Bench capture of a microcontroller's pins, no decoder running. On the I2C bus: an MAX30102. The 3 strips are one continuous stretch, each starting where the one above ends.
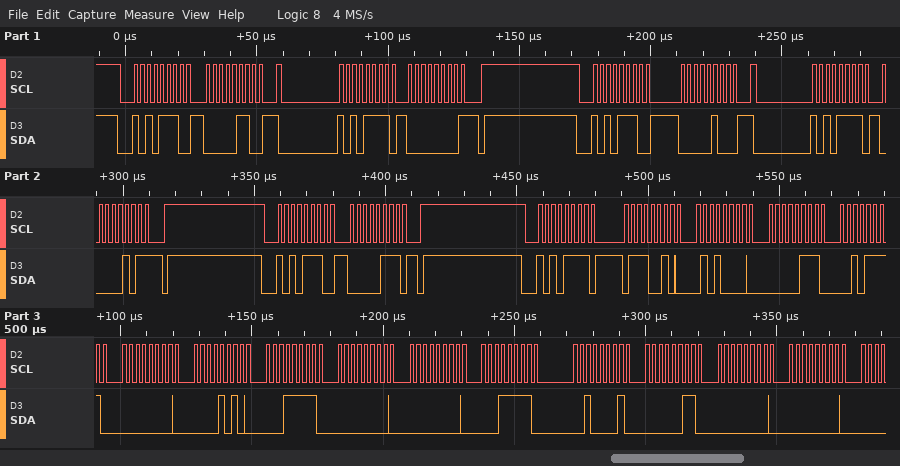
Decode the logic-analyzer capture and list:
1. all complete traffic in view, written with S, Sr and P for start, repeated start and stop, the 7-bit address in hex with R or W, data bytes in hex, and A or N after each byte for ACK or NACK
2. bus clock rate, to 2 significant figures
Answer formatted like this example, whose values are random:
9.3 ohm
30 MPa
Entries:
S 57W A 06 A Sr 57R A 00 N P S 57W A 04 A Sr 57R A 05 N P S 57W A 07 A P S 57R A 72 A 50 A 07 A 2F A 00 A 0A A 1F A 00 A 00 A 1F A 21 A 03 A 00 A 00 A
400 kHz
